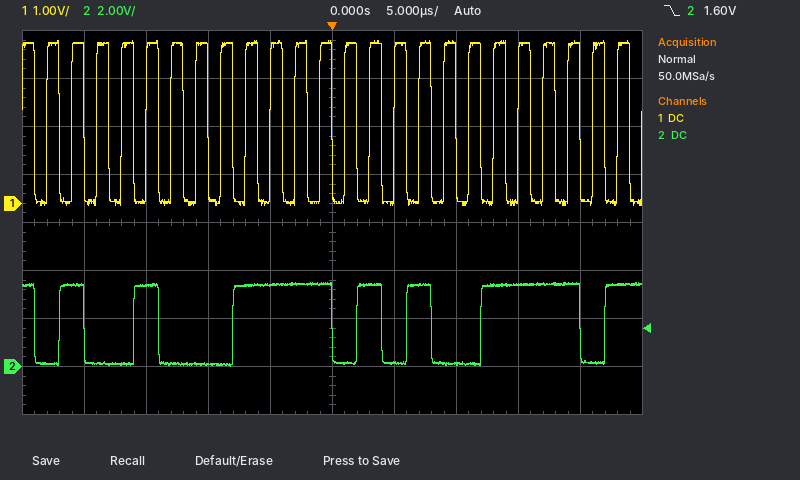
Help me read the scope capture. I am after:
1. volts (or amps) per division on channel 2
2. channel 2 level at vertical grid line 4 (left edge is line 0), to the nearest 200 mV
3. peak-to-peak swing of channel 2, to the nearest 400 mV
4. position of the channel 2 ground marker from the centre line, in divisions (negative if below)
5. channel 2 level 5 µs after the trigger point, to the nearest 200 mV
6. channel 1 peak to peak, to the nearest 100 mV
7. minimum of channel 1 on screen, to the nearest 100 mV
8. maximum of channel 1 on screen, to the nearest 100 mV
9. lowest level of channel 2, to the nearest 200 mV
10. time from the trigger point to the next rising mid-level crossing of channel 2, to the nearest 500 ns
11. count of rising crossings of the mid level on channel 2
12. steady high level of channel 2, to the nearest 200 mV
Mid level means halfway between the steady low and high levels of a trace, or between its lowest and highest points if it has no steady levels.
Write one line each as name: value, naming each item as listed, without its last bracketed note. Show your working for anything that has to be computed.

volts (or amps) per division on channel 2: 2 V
channel 2 level at vertical grid line 4 (left edge is line 0), to the nearest 200 mV: 3.4 V
peak-to-peak swing of channel 2, to the nearest 400 mV: 3.6 V
position of the channel 2 ground marker from the centre line, in divisions: -3.0 div
channel 2 level 5 µs after the trigger point, to the nearest 200 mV: 200 mV
channel 1 peak to peak, to the nearest 100 mV: 3.4 V − (0.0 V) = 3.4 V
minimum of channel 1 on screen, to the nearest 100 mV: 0.0 V
maximum of channel 1 on screen, to the nearest 100 mV: 3.4 V
lowest level of channel 2, to the nearest 200 mV: 0.0 V
time from the trigger point to the next rising mid-level crossing of channel 2, to the nearest 500 ns: 2.0 µs
count of rising crossings of the mid level on channel 2: 7
steady high level of channel 2, to the nearest 200 mV: 3.4 V
